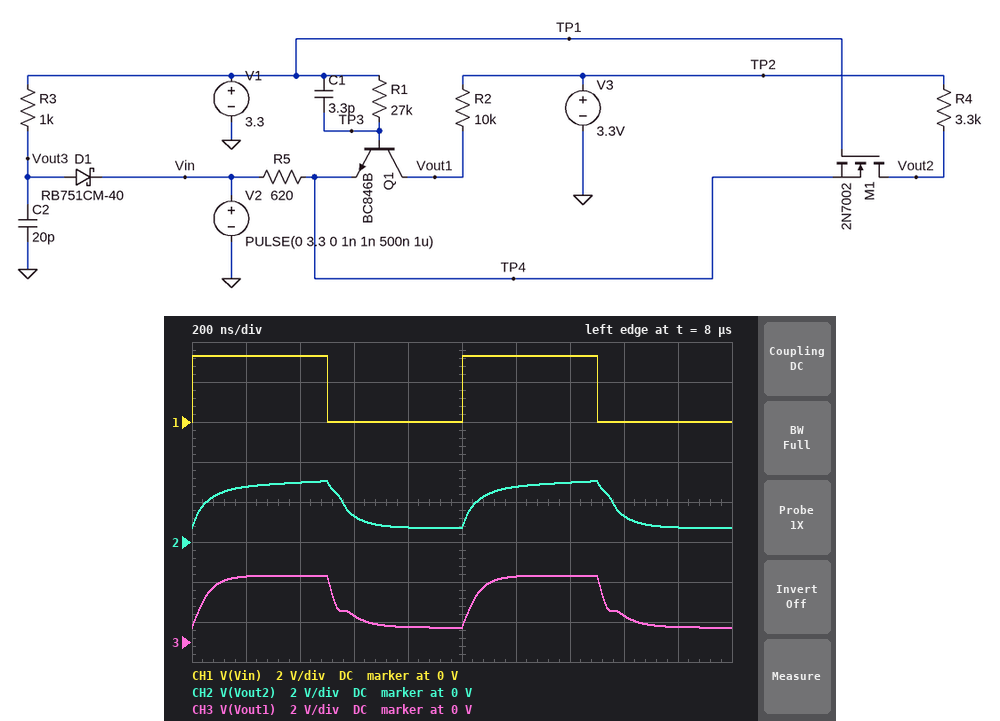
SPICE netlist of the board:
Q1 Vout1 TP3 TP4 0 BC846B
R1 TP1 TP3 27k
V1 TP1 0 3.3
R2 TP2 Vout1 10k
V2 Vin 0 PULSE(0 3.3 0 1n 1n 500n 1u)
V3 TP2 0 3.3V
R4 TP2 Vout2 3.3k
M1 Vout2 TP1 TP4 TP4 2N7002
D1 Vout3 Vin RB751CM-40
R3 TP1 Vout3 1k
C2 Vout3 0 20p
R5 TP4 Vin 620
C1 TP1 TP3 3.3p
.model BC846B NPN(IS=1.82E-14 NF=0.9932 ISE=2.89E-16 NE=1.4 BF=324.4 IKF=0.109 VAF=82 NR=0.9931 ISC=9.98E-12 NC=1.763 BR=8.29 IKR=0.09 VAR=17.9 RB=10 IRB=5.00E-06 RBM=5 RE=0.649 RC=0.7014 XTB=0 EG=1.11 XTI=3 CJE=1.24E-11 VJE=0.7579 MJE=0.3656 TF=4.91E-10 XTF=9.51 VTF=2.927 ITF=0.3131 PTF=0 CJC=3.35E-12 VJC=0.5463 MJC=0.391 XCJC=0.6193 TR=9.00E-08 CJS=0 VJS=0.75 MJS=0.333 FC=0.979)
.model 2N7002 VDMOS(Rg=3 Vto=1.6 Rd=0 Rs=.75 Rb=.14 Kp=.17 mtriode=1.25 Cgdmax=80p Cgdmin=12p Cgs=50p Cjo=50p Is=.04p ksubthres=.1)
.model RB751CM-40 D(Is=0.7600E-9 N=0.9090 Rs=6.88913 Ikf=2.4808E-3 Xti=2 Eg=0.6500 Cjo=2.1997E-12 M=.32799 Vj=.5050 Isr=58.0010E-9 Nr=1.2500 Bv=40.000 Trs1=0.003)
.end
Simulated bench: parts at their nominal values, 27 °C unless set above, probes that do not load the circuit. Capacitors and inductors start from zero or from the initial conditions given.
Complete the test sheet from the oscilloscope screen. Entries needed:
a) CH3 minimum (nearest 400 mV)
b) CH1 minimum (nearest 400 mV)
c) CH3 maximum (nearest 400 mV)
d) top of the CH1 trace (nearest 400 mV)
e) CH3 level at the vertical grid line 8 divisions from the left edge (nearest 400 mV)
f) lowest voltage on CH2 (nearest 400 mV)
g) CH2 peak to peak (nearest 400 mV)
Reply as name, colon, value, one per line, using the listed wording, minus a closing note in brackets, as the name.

CH3 minimum: 800 mV
CH1 minimum: 0 V
CH3 maximum: 3.2 V
top of the CH1 trace: 3.2 V
CH3 level at the vertical grid line 8 divisions from the left edge: 1.2 V
lowest voltage on CH2: 800 mV
CH2 peak to peak: 2.4 V
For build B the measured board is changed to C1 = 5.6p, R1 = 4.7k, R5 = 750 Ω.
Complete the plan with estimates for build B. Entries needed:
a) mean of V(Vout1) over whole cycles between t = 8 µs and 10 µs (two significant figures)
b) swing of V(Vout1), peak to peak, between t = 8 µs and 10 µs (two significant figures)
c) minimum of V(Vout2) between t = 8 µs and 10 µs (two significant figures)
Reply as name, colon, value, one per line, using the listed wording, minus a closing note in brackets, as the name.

mean of V(Vout1) over whole cycles between t = 8 µs and 10 µs: 2.1 V
swing of V(Vout1), peak to peak, between t = 8 µs and 10 µs: 2.3 V
minimum of V(Vout2) between t = 8 µs and 10 µs: 980 mV
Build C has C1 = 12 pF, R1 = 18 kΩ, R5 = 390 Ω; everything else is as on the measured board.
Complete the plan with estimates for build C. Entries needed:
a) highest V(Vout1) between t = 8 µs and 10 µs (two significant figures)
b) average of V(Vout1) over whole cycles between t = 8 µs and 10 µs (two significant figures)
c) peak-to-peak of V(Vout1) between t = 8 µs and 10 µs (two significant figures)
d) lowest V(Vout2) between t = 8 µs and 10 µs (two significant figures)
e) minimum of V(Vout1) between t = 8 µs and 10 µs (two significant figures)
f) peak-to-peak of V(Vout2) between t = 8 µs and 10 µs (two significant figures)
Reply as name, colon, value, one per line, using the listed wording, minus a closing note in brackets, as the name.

highest V(Vout1) between t = 8 µs and 10 µs: 3.3 V
average of V(Vout1) over whole cycles between t = 8 µs and 10 µs: 1.9 V
peak-to-peak of V(Vout1) between t = 8 µs and 10 µs: 2.8 V
lowest V(Vout2) between t = 8 µs and 10 µs: 490 mV
minimum of V(Vout1) between t = 8 µs and 10 µs: 500 mV
peak-to-peak of V(Vout2) between t = 8 µs and 10 µs: 2.6 V
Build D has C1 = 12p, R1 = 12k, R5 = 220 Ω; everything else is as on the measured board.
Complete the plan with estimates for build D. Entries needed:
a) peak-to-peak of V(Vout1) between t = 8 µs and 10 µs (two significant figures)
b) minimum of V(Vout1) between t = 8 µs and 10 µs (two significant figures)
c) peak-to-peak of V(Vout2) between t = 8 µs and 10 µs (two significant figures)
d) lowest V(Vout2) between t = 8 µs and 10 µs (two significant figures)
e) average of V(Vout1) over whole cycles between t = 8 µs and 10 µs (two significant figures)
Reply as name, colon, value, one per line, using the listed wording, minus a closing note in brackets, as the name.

peak-to-peak of V(Vout1) between t = 8 µs and 10 µs: 3.0 V
minimum of V(Vout1) between t = 8 µs and 10 µs: 320 mV
peak-to-peak of V(Vout2) between t = 8 µs and 10 µs: 2.8 V
lowest V(Vout2) between t = 8 µs and 10 µs: 310 mV
average of V(Vout1) over whole cycles between t = 8 µs and 10 µs: 1.8 V
